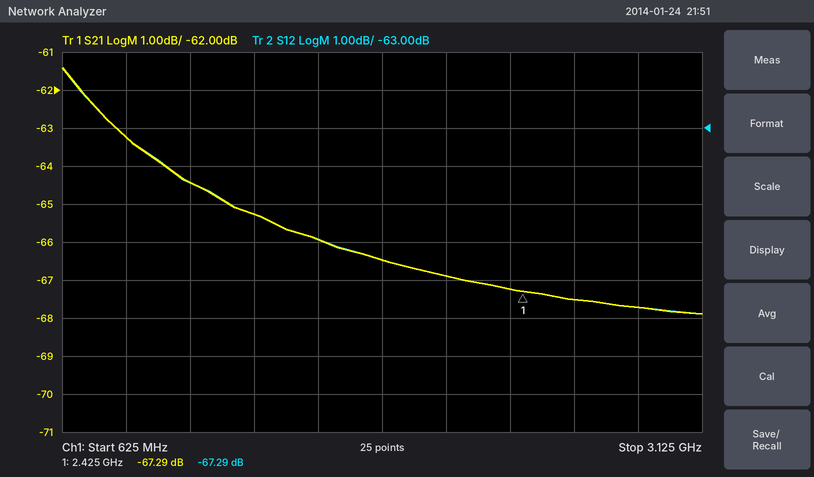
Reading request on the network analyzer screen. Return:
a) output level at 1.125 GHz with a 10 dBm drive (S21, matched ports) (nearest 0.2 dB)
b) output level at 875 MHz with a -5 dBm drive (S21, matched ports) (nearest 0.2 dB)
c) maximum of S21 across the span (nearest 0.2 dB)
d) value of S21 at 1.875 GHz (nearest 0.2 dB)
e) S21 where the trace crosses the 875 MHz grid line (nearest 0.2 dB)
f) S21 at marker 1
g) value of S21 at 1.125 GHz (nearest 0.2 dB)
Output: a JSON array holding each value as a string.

["-54.4 dBm", "-68.2 dBm", "-61.4 dB", "-66.4 dB", "-63.2 dB", "-67.29 dB", "-64.4 dB"]
